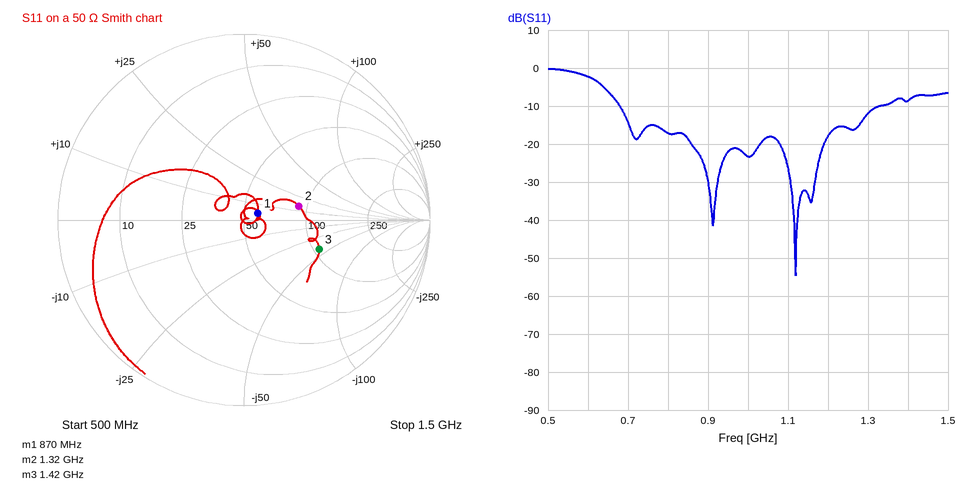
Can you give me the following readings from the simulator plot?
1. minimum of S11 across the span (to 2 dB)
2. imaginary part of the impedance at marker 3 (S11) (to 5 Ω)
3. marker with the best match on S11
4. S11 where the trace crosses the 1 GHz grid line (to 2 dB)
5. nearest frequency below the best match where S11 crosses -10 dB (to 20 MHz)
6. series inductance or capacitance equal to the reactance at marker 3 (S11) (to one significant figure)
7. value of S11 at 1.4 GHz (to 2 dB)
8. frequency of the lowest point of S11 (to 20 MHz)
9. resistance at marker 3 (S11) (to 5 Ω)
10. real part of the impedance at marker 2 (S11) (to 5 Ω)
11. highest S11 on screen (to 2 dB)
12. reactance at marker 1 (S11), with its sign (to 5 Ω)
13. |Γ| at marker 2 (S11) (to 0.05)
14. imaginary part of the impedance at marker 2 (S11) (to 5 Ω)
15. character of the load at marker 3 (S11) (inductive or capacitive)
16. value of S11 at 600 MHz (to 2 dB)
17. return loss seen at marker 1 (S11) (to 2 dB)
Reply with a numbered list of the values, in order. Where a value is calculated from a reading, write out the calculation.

1. -54 dB
2. -40 Ω
3. marker 1
4. -24 dB
5. 680 MHz
6. C = 1/(2π × 1.42 GHz × 40 Ω) ≈ 3 pF
7. -8 dB
8. 1.12 GHz
9. 105 Ω
10. 90 Ω
11. 0 dB
12. +5 Ω
13. 0.30
14. +15 Ω
15. capacitive
16. -2 dB
17. 22 dB
